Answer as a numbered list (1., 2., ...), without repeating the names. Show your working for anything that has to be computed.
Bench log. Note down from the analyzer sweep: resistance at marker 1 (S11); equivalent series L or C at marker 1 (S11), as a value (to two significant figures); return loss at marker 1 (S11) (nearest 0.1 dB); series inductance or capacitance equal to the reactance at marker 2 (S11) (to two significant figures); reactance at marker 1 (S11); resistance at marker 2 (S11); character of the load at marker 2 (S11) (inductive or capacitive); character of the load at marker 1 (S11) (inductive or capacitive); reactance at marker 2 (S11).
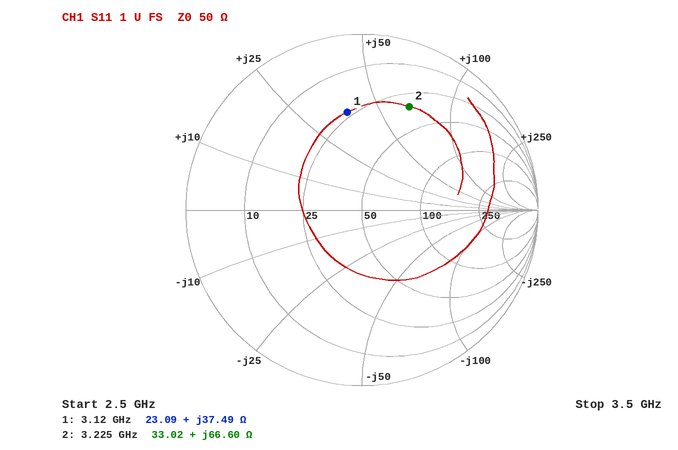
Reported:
1. 23.09 Ω
2. L = 37.49 Ω/(2π × 3.12 GHz) ≈ 1.9 nH
3. 5.0 dB
4. L = 66.6 Ω/(2π × 3.225 GHz) ≈ 3.3 nH
5. +37.49 Ω
6. 33.02 Ω
7. inductive
8. inductive
9. +66.60 Ω
